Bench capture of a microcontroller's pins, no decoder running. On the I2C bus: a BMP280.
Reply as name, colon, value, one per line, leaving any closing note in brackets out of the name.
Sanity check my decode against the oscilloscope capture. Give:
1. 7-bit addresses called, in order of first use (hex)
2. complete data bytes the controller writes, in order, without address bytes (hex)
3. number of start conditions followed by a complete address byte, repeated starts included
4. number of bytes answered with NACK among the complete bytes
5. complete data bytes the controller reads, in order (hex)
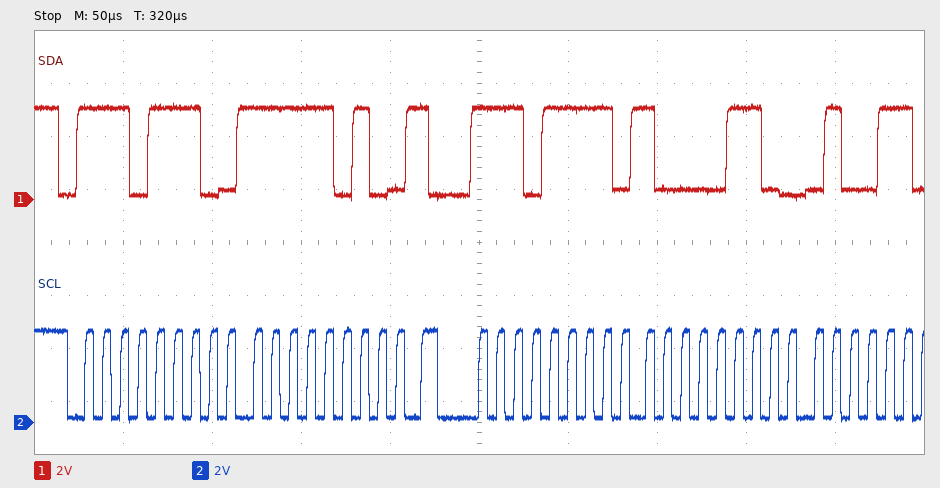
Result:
7-bit addresses called, in order of first use: 0x77
complete data bytes the controller writes, in order, without address bytes: FA
number of start conditions followed by a complete address byte, repeated starts included: 2
number of bytes answered with NACK among the complete bytes: 0
complete data bytes the controller reads, in order: 86
